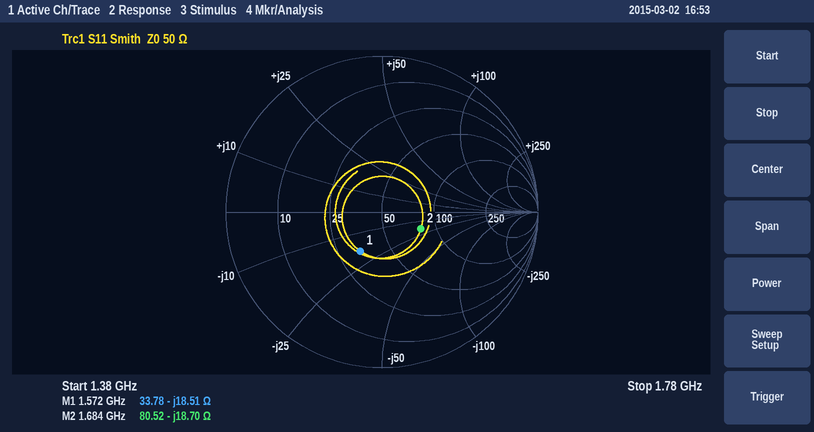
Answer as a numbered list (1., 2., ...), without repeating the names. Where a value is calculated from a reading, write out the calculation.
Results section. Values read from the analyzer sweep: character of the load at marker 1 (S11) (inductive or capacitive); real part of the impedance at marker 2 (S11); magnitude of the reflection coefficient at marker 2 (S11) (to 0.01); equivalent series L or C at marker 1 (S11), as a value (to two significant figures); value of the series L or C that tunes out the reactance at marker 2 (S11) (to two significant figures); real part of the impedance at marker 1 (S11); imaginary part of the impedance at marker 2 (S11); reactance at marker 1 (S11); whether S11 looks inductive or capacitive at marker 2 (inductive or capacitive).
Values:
1. capacitive
2. 80.52 Ω
3. 0.27
4. C = 1/(2π × 1.572 GHz × 18.51 Ω) ≈ 5.5 pF
5. L = 18.7 Ω/(2π × 1.684 GHz) ≈ 1.8 nH
6. 33.78 Ω
7. -18.70 Ω
8. -18.51 Ω
9. capacitive
